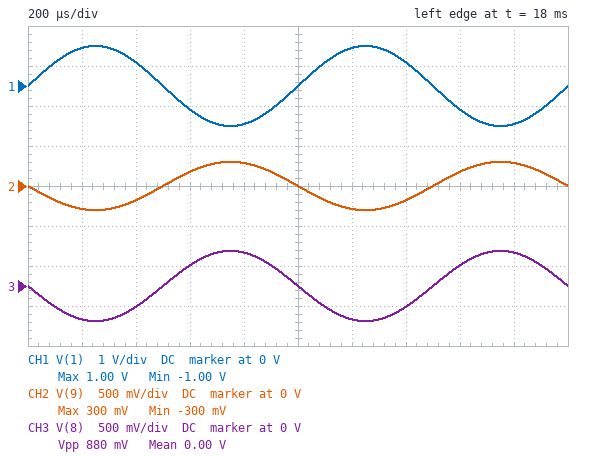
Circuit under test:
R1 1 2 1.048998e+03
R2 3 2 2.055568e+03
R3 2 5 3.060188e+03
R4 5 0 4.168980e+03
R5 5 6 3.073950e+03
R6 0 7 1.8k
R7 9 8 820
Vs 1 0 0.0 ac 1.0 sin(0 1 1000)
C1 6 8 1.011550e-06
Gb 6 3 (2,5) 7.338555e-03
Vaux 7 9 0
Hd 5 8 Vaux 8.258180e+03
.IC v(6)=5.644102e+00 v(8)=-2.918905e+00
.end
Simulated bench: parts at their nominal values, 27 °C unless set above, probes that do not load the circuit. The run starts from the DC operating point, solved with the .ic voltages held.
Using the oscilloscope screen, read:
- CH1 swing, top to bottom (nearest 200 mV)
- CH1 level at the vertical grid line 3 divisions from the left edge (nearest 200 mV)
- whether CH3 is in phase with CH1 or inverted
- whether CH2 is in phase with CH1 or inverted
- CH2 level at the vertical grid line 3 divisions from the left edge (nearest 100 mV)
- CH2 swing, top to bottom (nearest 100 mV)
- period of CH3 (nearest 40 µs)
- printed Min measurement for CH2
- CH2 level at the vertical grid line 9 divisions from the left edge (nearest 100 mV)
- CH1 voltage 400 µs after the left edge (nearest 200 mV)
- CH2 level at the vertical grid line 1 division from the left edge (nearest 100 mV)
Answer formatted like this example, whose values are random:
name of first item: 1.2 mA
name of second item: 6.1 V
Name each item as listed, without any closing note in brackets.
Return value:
CH1 swing, top to bottom: 2.0 V
CH1 level at the vertical grid line 3 divisions from the left edge: -600 mV
whether CH3 is in phase with CH1 or inverted: inverted
whether CH2 is in phase with CH1 or inverted: inverted
CH2 level at the vertical grid line 3 divisions from the left edge: 200 mV
CH2 swing, top to bottom: 600 mV
period of CH3: 1.00 ms
printed Min measurement for CH2: -300 mV
CH2 level at the vertical grid line 9 divisions from the left edge: 300 mV
CH1 voltage 400 µs after the left edge: 600 mV
CH2 level at the vertical grid line 1 division from the left edge: -300 mV
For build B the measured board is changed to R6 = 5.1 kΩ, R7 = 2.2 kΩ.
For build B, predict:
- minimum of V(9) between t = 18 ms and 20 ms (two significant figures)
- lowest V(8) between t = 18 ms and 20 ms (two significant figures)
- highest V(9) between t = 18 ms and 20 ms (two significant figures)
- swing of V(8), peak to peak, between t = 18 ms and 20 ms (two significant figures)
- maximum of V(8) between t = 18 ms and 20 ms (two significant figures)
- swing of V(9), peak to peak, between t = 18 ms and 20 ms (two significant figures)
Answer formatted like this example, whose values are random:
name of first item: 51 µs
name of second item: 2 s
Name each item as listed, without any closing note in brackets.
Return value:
minimum of V(9) between t = 18 ms and 20 ms: -20 V
lowest V(8) between t = 18 ms and 20 ms: -28 V
highest V(9) between t = 18 ms and 20 ms: 20 V
swing of V(8), peak to peak, between t = 18 ms and 20 ms: 56 V
maximum of V(8) between t = 18 ms and 20 ms: 28 V
swing of V(9), peak to peak, between t = 18 ms and 20 ms: 39 V
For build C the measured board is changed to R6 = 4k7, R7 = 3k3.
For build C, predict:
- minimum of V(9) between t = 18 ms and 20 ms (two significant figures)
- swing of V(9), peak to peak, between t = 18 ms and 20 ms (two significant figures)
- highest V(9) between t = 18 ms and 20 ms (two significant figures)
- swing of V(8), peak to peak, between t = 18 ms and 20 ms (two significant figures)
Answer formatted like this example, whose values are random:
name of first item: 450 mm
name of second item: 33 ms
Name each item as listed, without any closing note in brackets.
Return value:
minimum of V(9) between t = 18 ms and 20 ms: -7.9 V
swing of V(9), peak to peak, between t = 18 ms and 20 ms: 16 V
highest V(9) between t = 18 ms and 20 ms: 7.9 V
swing of V(8), peak to peak, between t = 18 ms and 20 ms: 27 V
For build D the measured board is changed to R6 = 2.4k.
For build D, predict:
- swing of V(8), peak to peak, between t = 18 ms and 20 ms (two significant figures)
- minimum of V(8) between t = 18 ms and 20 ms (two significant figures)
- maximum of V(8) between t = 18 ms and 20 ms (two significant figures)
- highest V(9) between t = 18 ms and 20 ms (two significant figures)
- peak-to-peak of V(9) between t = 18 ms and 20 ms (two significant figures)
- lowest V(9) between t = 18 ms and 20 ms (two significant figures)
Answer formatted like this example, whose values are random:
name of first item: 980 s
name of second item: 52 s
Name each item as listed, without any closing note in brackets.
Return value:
swing of V(8), peak to peak, between t = 18 ms and 20 ms: 1.2 V
minimum of V(8) between t = 18 ms and 20 ms: -620 mV
maximum of V(8) between t = 18 ms and 20 ms: 620 mV
highest V(9) between t = 18 ms and 20 ms: 460 mV
peak-to-peak of V(9) between t = 18 ms and 20 ms: 920 mV
lowest V(9) between t = 18 ms and 20 ms: -460 mV
